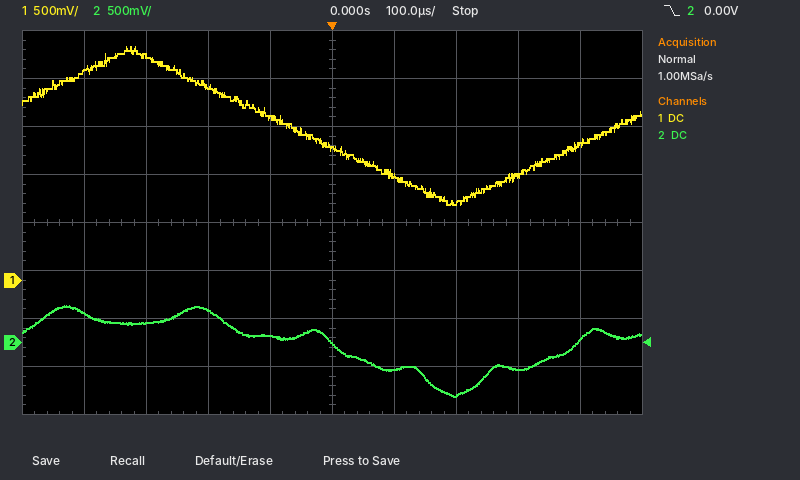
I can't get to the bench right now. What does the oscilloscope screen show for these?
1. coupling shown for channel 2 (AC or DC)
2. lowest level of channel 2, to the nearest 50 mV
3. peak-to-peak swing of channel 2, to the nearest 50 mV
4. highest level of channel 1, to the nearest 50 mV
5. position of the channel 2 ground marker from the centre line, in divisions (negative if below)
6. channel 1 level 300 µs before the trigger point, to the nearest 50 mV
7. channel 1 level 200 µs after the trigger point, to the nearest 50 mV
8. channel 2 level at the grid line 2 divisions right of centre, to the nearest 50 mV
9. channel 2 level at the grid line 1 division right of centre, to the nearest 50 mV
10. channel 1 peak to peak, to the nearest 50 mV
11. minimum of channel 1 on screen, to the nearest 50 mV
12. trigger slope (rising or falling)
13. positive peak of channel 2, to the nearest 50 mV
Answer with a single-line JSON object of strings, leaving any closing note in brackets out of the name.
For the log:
{"coupling shown for channel 2": "DC", "lowest level of channel 2, to the nearest 50 mV": "-550 mV", "peak-to-peak swing of channel 2, to the nearest 50 mV": "950 mV", "highest level of channel 1, to the nearest 50 mV": "2.45 V", "position of the channel 2 ground marker from the centre line, in divisions": "-2.5 div", "channel 1 level 300 µs before the trigger point, to the nearest 50 mV": "2.35 V", "channel 1 level 200 µs after the trigger point, to the nearest 50 mV": "800 mV", "channel 2 level at the grid line 2 divisions right of centre, to the nearest 50 mV": "-550 mV", "channel 2 level at the grid line 1 division right of centre, to the nearest 50 mV": "-300 mV", "channel 1 peak to peak, to the nearest 50 mV": "1.65 V", "minimum of channel 1 on screen, to the nearest 50 mV": "800 mV", "trigger slope": "falling", "positive peak of channel 2, to the nearest 50 mV": "400 mV"}
